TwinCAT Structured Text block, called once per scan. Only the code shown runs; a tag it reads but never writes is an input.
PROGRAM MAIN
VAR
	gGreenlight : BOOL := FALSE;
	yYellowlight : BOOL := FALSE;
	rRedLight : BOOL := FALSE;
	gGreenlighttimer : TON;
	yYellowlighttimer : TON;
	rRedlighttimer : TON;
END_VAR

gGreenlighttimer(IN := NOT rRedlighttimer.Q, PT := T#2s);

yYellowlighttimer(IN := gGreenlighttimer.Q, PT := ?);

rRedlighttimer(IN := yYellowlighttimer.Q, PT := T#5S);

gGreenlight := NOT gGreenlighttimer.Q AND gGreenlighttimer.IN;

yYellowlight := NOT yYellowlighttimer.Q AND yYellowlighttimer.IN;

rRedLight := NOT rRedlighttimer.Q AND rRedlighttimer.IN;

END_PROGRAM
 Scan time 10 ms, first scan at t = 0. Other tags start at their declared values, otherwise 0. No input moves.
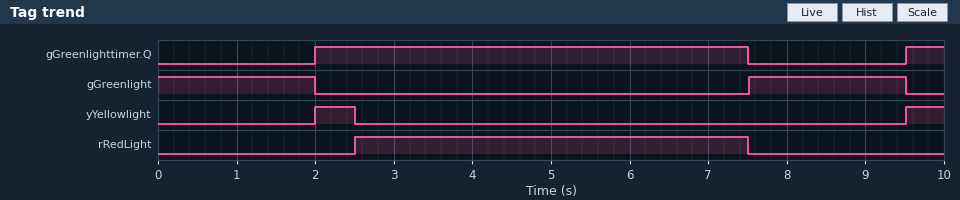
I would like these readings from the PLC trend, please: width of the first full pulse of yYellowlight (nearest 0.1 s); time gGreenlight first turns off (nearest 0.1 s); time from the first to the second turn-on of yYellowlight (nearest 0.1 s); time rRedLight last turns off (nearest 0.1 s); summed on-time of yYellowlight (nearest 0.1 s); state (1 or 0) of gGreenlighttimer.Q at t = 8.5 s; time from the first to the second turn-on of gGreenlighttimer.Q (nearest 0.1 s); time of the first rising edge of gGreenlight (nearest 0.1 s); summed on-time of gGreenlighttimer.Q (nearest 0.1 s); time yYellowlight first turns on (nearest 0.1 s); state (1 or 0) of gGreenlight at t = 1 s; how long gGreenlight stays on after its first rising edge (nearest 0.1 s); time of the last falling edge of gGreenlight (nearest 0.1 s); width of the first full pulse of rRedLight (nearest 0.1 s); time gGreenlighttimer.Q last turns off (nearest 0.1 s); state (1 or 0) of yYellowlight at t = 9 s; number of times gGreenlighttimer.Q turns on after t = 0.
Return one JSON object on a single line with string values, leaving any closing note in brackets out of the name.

{"width of the first full pulse of yYellowlight": "0.5 s", "time gGreenlight first turns off": "2.0 s", "time from the first to the second turn-on of yYellowlight": "7.5 s", "time rRedLight last turns off": "7.5 s", "summed on-time of yYellowlight": "1.0 s", "state (1 or 0) of gGreenlighttimer.Q at t = 8.5 s": "0", "time from the first to the second turn-on of gGreenlighttimer.Q": "7.5 s", "time of the first rising edge of gGreenlight": "7.5 s", "summed on-time of gGreenlighttimer.Q": "6.0 s", "time yYellowlight first turns on": "2.0 s", "state (1 or 0) of gGreenlight at t = 1 s": "1", "how long gGreenlight stays on after its first rising edge": "2.0 s", "time of the last falling edge of gGreenlight": "9.5 s", "width of the first full pulse of rRedLight": "5.0 s", "time gGreenlighttimer.Q last turns off": "7.5 s", "state (1 or 0) of yYellowlight at t = 9 s": "0", "number of times gGreenlighttimer.Q turns on after t = 0": "2"}
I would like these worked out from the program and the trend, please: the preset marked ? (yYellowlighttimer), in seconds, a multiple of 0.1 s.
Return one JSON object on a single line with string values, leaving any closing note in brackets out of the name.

{"the preset marked ? (yYellowlighttimer), in seconds, a multiple of 0.1 s": "0.5 s"}
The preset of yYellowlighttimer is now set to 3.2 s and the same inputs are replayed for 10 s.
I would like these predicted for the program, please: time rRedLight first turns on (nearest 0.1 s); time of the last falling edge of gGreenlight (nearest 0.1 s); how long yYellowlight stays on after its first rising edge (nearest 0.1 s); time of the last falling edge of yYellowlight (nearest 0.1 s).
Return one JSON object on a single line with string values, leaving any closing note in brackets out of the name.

{"time rRedLight first turns on": "5.2 s", "time of the last falling edge of gGreenlight": "2.0 s", "how long yYellowlight stays on after its first rising edge": "3.2 s", "time of the last falling edge of yYellowlight": "5.2 s"}
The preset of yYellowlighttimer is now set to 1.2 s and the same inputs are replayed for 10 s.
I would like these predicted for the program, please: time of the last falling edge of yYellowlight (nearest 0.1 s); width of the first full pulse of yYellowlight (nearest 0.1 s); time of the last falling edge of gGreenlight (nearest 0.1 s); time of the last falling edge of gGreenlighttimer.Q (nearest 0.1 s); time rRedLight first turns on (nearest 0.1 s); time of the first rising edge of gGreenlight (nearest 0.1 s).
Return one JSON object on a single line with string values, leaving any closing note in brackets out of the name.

{"time of the last falling edge of yYellowlight": "3.2 s", "width of the first full pulse of yYellowlight": "1.2 s", "time of the last falling edge of gGreenlight": "2.0 s", "time of the last falling edge of gGreenlighttimer.Q": "8.2 s", "time rRedLight first turns on": "3.2 s", "time of the first rising edge of gGreenlight": "8.2 s"}
